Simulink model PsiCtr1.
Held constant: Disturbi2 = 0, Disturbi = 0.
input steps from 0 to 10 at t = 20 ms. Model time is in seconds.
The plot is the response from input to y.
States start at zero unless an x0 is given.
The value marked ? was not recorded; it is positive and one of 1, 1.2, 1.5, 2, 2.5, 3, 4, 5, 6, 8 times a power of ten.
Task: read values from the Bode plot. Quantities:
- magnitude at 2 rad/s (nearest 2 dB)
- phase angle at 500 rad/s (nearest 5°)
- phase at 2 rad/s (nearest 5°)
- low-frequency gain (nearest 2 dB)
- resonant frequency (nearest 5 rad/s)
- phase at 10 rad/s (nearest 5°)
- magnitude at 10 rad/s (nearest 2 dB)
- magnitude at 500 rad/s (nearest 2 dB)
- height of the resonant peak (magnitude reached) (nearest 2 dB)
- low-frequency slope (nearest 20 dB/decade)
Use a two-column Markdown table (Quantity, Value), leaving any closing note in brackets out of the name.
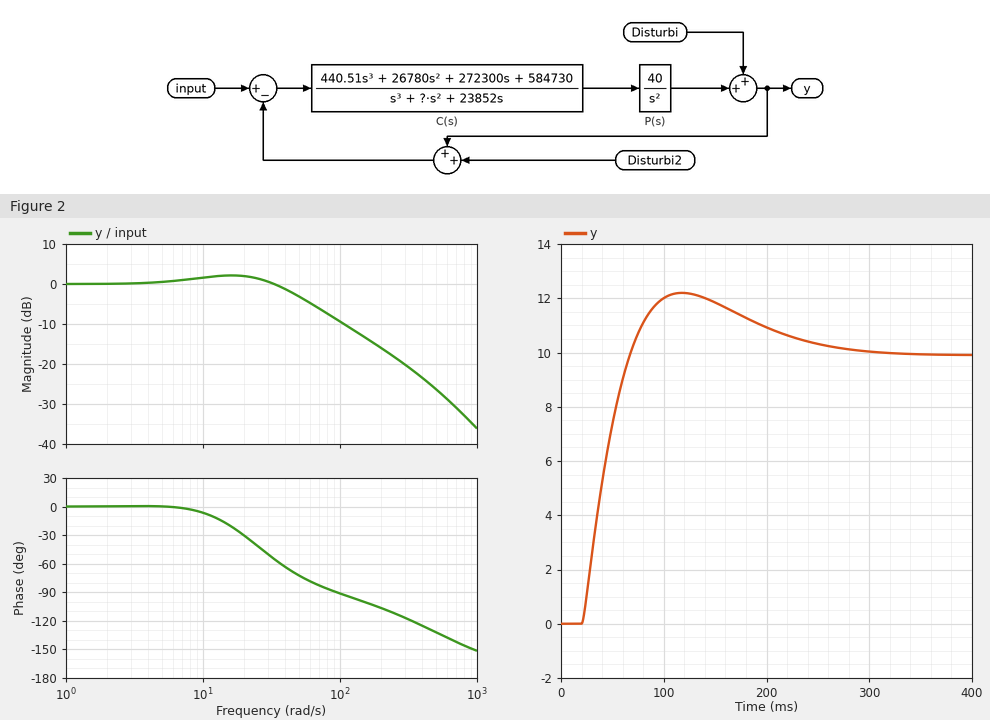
| Quantity | Value |
|---|---|
| magnitude at 2 rad/s | 0 dB |
| phase angle at 500 rad/s | -130° |
| phase at 2 rad/s | 0° |
| low-frequency gain | 0 dB |
| resonant frequency | 15 rad/s |
| phase at 10 rad/s | -5° |
| magnitude at 10 rad/s | 2 dB |
| magnitude at 500 rad/s | -26 dB |
| height of the resonant peak (magnitude reached) | 2 dB |
| low-frequency slope | 0 dB/decade |
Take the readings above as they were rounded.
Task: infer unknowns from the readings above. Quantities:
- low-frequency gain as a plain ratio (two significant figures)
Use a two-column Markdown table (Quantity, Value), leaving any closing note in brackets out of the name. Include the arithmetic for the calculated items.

| Quantity | Value |
|---|---|
| low-frequency gain as a plain ratio | 10^(0 / 20) = 1.0 |
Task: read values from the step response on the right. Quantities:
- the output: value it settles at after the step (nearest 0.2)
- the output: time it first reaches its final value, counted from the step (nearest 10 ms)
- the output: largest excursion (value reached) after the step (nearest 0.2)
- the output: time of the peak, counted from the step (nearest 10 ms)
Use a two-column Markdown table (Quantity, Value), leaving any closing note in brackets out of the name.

| Quantity | Value |
|---|---|
| the output: value it settles at after the step | 10.0 |
| the output: time it first reaches its final value, counted from the step | 50 ms |
| the output: largest excursion (value reached) after the step | 12.2 |
| the output: time of the peak, counted from the step | 100 ms |
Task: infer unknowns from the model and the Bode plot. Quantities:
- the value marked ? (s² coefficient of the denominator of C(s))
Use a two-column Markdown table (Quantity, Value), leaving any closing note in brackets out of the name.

| Quantity | Value |
|---|---|
| the value marked ? (s² coefficient of the denominator of C(s)) | 600 |
